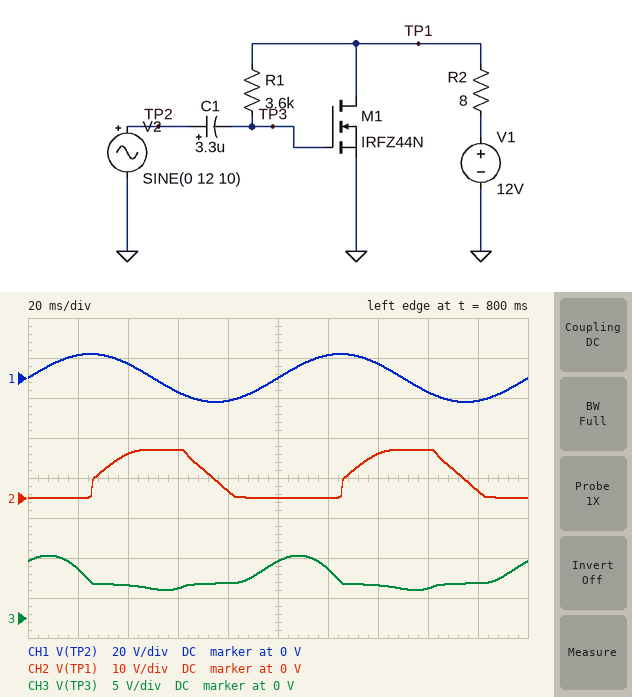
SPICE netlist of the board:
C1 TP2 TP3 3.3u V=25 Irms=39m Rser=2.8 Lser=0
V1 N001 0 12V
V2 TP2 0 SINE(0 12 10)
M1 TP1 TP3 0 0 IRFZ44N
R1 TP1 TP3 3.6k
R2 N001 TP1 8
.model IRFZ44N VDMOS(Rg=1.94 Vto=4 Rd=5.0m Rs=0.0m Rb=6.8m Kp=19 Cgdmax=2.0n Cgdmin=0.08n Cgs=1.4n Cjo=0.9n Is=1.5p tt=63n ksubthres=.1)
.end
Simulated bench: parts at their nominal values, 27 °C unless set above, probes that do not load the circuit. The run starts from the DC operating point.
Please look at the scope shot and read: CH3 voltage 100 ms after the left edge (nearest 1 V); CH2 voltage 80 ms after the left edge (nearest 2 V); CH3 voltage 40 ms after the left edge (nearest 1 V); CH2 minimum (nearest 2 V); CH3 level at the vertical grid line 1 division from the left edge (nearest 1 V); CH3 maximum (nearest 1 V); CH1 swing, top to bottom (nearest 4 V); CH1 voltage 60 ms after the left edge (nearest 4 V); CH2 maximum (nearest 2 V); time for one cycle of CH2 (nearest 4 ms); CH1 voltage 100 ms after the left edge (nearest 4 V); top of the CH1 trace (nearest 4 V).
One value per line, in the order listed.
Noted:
7 V
2 V
4 V
0 V
6 V
8 V
24 V
-8 V
12 V
100 ms
0 V
12 V
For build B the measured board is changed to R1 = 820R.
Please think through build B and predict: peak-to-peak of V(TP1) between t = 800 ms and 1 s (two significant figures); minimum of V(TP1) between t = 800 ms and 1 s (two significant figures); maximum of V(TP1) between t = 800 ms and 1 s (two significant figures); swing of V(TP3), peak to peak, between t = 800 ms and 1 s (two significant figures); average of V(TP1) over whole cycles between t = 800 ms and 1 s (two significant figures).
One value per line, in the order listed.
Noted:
4.0 V
2.3 V
6.3 V
88 mV
4.3 V
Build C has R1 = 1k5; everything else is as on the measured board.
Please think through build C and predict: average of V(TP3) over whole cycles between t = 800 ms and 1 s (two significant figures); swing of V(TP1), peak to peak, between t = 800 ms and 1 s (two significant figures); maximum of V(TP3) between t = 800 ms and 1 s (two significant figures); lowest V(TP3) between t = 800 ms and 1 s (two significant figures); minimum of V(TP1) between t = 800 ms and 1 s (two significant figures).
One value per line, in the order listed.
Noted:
4.3 V
7.3 V
4.4 V
4.2 V
650 mV
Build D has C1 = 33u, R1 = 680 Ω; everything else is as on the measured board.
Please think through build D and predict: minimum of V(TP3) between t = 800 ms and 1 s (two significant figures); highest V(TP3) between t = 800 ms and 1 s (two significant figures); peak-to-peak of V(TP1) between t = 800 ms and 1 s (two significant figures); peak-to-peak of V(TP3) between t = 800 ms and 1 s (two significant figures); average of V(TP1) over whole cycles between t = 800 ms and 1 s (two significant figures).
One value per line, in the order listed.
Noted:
-980 mV
12 V
12 V
13 V
5.3 V
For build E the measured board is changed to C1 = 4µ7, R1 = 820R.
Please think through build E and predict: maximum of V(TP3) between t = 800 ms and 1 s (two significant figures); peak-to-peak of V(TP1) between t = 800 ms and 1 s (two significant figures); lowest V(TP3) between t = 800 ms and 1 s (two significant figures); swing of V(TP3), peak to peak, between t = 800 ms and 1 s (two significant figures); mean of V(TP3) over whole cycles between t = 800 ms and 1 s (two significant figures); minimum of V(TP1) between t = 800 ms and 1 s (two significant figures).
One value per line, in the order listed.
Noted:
4.4 V
5.7 V
4.2 V
130 mV
4.3 V
1.5 V
